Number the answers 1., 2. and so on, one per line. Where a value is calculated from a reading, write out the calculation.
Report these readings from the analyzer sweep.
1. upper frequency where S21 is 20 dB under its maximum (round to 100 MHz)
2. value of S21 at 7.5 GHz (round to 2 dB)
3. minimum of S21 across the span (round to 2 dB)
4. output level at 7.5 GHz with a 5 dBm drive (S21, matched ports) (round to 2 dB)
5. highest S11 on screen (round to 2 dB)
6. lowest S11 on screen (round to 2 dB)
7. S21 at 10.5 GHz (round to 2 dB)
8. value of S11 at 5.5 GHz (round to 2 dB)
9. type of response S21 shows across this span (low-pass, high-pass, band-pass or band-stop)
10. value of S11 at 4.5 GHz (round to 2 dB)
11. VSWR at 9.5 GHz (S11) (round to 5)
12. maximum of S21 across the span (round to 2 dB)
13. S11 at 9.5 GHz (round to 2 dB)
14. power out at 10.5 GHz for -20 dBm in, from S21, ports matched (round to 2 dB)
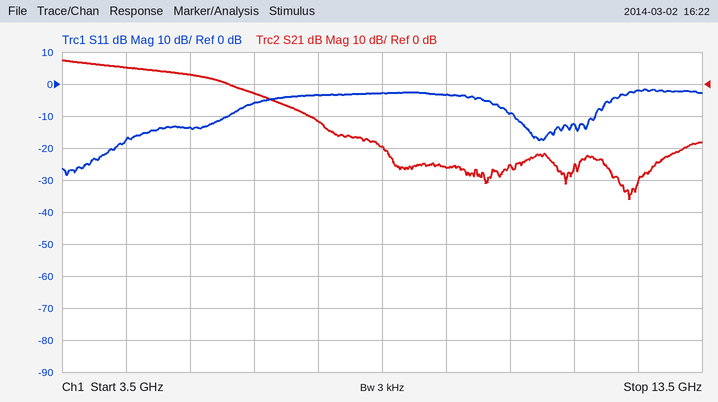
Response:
1. 7.6 GHz
2. -12 dB
3. -36 dB
4. 5 dBm + (-12 dB) = -6 dBm
5. -2 dB
6. -28 dB
7. -26 dB
8. -14 dB
9. low-pass
10. -18 dB
11. |Γ| = 10^(-4/20) = 0.6310; VSWR = (1 + 0.6310)/(1 − 0.6310) ≈ 4.42, so 5 to the nearest 5
12. 8 dB
13. -4 dB
14. -20 dBm + (-26 dB) = -46 dBm
